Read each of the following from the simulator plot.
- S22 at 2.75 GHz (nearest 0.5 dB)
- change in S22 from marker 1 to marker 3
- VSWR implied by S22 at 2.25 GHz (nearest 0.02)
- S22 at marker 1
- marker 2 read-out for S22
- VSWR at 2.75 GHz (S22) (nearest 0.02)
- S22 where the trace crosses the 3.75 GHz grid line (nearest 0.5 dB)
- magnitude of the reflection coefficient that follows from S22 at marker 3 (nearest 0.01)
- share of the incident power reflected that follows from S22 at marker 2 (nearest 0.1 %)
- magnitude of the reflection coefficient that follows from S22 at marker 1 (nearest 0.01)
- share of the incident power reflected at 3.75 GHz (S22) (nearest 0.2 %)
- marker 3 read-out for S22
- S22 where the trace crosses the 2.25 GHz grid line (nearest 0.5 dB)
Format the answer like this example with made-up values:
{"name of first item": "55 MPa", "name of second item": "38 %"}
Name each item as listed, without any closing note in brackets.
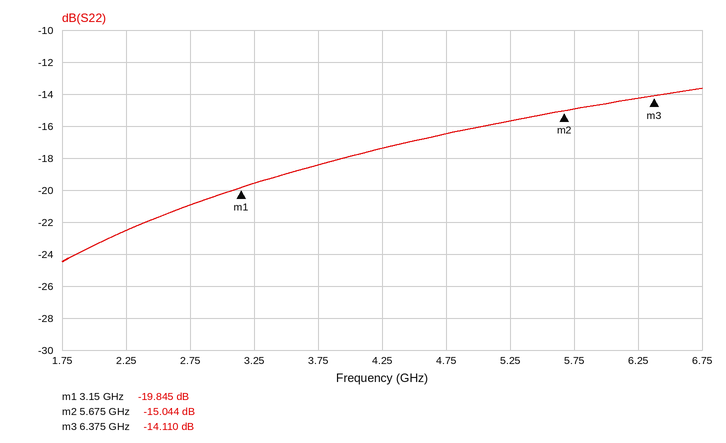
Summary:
{"S22 at 2.75 GHz": "-21.0 dB", "change in S22 from marker 1 to marker 3": "5.735 dB", "VSWR implied by S22 at 2.25 GHz": "1.16", "S22 at marker 1": "-19.845 dB", "marker 2 read-out for S22": "-15.044 dB", "VSWR at 2.75 GHz (S22)": "1.20", "S22 where the trace crosses the 3.75 GHz grid line": "-18.5 dB", "magnitude of the reflection coefficient that follows from S22 at marker 3": "0.20", "share of the incident power reflected that follows from S22 at marker 2": "3.1 %", "magnitude of the reflection coefficient that follows from S22 at marker 1": "0.10", "share of the incident power reflected at 3.75 GHz (S22)": "1.4 %", "marker 3 read-out for S22": "-14.110 dB", "S22 where the trace crosses the 2.25 GHz grid line": "-22.5 dB"}
